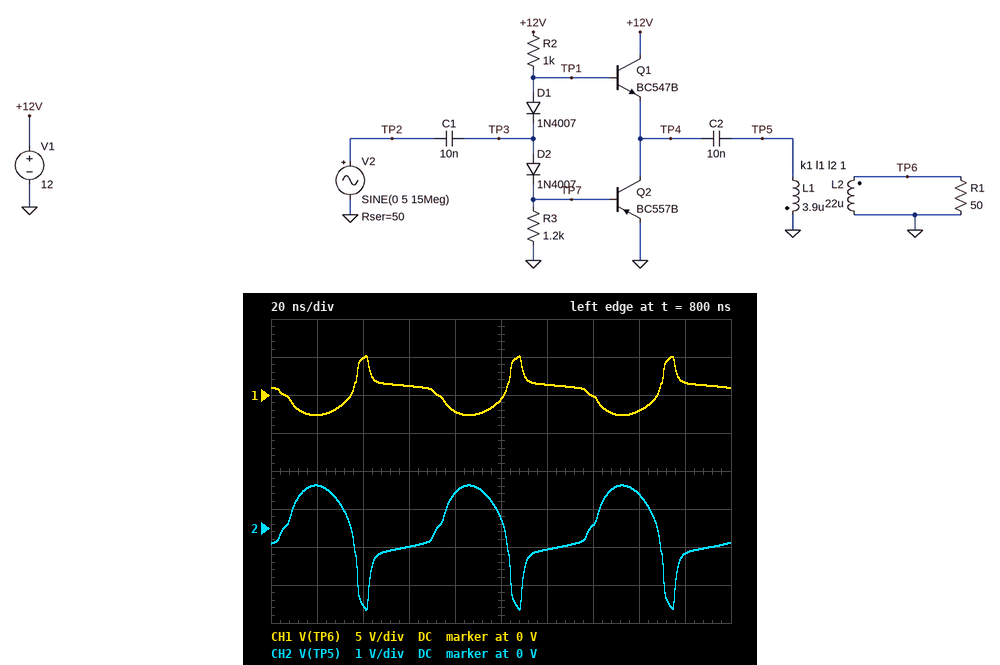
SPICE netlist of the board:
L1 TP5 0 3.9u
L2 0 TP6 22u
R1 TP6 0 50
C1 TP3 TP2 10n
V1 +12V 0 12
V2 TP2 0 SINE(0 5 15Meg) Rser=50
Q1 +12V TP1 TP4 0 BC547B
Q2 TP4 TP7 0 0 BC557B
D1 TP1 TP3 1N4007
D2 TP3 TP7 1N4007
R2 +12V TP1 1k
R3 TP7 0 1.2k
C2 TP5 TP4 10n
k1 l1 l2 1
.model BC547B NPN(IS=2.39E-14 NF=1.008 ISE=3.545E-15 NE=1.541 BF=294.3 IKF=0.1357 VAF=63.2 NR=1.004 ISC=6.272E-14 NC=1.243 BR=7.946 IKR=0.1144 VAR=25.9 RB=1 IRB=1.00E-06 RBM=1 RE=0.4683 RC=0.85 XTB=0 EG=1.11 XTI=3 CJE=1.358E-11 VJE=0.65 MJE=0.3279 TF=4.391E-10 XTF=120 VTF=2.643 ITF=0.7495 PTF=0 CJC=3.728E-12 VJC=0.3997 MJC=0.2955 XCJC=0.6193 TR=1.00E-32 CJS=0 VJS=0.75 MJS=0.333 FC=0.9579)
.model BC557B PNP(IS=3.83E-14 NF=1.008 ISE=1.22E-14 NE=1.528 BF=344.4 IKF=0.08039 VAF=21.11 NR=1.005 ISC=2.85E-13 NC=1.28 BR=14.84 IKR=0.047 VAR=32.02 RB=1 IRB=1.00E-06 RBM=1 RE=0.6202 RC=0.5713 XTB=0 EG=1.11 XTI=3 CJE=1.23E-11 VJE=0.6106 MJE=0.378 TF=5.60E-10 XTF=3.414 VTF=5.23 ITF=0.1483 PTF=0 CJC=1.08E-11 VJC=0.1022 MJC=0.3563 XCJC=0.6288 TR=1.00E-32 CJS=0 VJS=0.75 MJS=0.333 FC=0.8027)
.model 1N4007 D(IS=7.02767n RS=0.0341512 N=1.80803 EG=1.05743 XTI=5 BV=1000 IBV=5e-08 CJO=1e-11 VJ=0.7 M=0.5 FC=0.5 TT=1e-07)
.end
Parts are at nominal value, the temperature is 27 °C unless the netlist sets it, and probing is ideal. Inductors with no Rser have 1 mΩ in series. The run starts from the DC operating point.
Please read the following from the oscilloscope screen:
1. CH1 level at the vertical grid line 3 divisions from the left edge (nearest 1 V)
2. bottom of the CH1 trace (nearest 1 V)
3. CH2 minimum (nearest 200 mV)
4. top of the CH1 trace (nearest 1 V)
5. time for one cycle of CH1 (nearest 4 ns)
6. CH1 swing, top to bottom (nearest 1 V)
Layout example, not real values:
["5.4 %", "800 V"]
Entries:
["1 V", "-3 V", "-2.2 V", "5 V", "68 ns", "8 V"]
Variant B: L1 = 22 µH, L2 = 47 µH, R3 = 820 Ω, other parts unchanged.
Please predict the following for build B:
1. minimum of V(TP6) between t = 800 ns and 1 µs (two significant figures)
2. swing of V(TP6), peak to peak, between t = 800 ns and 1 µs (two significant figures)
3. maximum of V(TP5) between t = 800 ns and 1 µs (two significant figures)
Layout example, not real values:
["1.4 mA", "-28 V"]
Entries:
["-4.0 V", "9.1 V", "2.8 V"]
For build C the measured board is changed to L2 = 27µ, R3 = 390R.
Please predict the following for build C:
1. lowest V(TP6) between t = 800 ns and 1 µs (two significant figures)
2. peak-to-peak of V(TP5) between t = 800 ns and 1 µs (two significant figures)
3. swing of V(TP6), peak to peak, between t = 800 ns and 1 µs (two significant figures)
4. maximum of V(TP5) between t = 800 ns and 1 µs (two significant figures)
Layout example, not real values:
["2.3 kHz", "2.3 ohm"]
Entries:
["-3.2 V", "3.2 V", "8.3 V", "1.2 V"]
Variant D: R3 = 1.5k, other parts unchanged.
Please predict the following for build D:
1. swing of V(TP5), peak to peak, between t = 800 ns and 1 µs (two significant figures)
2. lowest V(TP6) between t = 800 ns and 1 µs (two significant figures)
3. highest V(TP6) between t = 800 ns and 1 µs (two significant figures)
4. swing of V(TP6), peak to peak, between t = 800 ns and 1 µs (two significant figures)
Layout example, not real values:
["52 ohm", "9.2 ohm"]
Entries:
["3.2 V", "-2.5 V", "5.0 V", "7.6 V"]
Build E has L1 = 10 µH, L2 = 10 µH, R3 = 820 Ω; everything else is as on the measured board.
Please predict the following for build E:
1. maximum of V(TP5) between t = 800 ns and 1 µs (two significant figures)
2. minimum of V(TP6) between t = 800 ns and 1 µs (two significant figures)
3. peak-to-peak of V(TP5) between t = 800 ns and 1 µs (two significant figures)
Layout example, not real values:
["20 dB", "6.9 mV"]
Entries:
["3.9 V", "-3.9 V", "7.8 V"]
